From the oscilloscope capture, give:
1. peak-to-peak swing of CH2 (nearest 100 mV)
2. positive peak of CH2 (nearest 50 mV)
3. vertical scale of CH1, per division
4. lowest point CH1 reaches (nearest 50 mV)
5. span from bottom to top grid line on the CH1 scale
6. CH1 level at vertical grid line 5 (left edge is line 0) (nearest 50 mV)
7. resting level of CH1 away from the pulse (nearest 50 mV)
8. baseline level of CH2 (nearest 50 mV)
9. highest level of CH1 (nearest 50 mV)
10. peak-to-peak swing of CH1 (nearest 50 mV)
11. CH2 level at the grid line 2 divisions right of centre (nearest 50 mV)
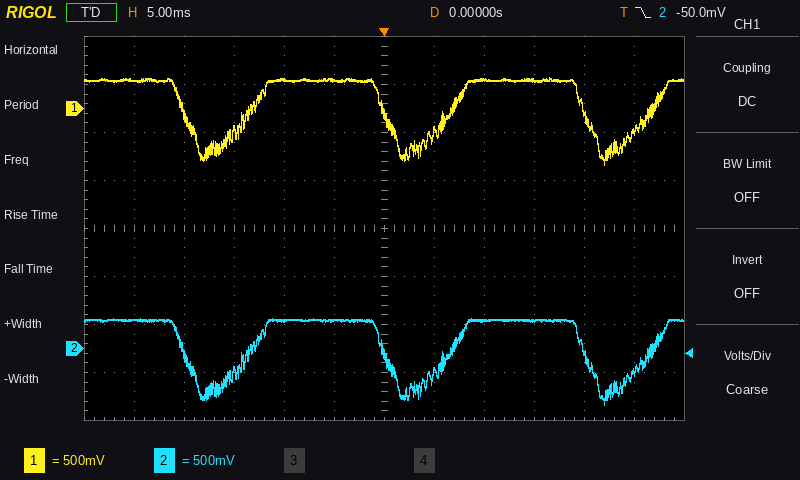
900 mV
300 mV
500 mV
-600 mV
4 V
300 mV
300 mV
300 mV
300 mV
900 mV
300 mV
